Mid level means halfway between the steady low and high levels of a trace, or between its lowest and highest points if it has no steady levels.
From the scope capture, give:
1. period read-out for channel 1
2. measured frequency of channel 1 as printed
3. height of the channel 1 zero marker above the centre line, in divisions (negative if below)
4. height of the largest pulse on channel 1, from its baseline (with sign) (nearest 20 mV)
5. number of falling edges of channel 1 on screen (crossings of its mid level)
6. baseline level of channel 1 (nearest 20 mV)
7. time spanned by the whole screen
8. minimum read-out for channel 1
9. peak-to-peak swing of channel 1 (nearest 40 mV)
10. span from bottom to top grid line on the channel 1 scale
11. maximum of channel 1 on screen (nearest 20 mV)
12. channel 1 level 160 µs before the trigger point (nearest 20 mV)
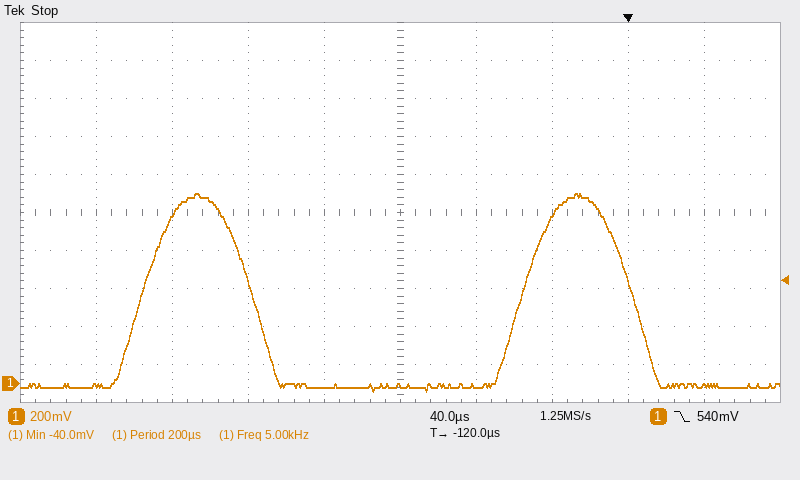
200 µs
5.00 kHz
-4.5 div
+1.02 V
2
-20 mV
400 µs
-40.0 mV
1.04 V
2 V
1.00 V
-20 mV
